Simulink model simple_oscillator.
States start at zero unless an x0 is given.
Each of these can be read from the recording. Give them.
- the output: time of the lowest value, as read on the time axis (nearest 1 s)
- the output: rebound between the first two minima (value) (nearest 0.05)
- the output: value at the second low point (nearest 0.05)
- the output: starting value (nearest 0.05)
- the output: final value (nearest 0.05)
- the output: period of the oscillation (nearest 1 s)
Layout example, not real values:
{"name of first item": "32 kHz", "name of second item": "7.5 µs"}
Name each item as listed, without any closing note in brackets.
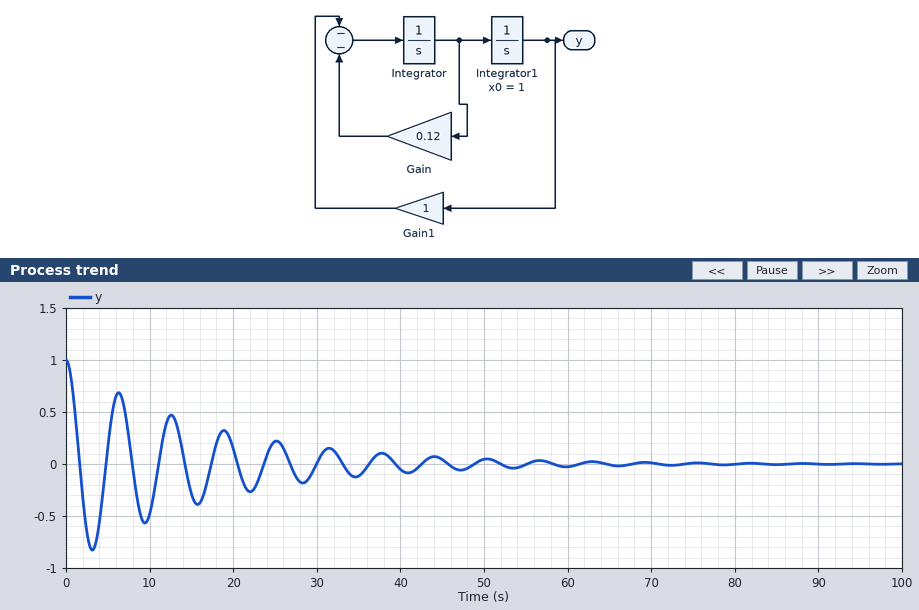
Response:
{"the output: time of the lowest value, as read on the time axis": "3 s", "the output: rebound between the first two minima (value)": "0.70", "the output: value at the second low point": "-0.55", "the output: starting value": "1.00", "the output: final value": "0.00", "the output: period of the oscillation": "6 s"}
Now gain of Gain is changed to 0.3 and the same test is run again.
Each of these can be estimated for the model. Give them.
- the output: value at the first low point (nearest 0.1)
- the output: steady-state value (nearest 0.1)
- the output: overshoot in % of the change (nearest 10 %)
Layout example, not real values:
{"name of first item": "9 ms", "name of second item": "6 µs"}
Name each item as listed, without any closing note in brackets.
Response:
{"the output: value at the first low point": "-0.6", "the output: steady-state value": "0.0", "the output: overshoot in % of the change": "60 %"}
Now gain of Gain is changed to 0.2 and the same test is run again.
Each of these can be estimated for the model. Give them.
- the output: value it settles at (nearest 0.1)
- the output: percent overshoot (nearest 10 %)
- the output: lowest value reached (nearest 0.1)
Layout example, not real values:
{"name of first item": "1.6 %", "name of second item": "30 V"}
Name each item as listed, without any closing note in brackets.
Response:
{"the output: value it settles at": "0.0", "the output: percent overshoot": "70 %", "the output: lowest value reached": "-0.7"}
